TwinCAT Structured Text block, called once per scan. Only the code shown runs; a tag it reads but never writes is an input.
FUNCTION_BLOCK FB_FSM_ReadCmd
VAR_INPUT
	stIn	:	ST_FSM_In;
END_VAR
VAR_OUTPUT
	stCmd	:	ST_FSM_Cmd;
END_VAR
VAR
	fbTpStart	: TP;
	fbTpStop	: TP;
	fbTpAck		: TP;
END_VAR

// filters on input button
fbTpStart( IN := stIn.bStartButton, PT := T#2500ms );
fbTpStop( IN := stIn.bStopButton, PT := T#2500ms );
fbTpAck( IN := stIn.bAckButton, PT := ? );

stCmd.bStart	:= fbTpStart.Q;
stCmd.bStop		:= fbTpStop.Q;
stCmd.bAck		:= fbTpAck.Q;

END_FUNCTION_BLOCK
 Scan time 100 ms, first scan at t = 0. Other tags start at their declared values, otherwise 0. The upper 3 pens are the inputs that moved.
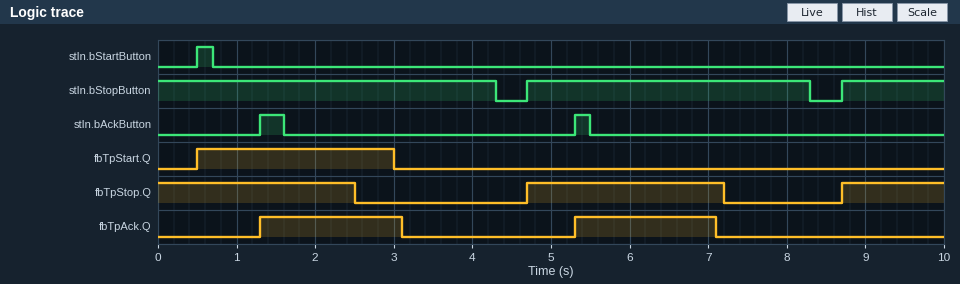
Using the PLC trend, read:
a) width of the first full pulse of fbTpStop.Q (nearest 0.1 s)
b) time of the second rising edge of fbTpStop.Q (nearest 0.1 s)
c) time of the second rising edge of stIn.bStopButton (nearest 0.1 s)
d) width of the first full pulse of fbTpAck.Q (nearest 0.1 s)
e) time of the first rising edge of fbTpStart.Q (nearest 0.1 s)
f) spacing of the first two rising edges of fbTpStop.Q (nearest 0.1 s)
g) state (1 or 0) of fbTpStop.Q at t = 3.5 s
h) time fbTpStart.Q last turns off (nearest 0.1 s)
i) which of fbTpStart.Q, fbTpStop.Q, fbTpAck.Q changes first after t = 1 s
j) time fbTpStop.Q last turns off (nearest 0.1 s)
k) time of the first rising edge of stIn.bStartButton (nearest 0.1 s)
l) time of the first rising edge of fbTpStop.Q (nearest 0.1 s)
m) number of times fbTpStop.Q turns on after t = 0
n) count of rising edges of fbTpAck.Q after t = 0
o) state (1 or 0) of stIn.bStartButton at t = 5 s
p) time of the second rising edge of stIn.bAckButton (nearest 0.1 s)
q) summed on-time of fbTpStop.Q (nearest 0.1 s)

2.5 s
8.7 s
8.7 s
1.8 s
0.5 s
4.0 s
0
3.0 s
fbTpAck.Q
7.2 s
0.5 s
4.7 s
2
2
0
5.3 s
6.3 s
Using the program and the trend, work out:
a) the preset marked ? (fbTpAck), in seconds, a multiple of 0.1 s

1.8 s
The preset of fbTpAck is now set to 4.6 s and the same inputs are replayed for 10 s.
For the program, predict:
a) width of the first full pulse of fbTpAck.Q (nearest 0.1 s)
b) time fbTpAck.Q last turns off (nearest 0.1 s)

4.6 s
5.9 s
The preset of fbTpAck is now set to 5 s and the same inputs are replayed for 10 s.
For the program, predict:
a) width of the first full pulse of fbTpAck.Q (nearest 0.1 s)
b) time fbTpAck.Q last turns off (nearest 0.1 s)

5.0 s
6.3 s
